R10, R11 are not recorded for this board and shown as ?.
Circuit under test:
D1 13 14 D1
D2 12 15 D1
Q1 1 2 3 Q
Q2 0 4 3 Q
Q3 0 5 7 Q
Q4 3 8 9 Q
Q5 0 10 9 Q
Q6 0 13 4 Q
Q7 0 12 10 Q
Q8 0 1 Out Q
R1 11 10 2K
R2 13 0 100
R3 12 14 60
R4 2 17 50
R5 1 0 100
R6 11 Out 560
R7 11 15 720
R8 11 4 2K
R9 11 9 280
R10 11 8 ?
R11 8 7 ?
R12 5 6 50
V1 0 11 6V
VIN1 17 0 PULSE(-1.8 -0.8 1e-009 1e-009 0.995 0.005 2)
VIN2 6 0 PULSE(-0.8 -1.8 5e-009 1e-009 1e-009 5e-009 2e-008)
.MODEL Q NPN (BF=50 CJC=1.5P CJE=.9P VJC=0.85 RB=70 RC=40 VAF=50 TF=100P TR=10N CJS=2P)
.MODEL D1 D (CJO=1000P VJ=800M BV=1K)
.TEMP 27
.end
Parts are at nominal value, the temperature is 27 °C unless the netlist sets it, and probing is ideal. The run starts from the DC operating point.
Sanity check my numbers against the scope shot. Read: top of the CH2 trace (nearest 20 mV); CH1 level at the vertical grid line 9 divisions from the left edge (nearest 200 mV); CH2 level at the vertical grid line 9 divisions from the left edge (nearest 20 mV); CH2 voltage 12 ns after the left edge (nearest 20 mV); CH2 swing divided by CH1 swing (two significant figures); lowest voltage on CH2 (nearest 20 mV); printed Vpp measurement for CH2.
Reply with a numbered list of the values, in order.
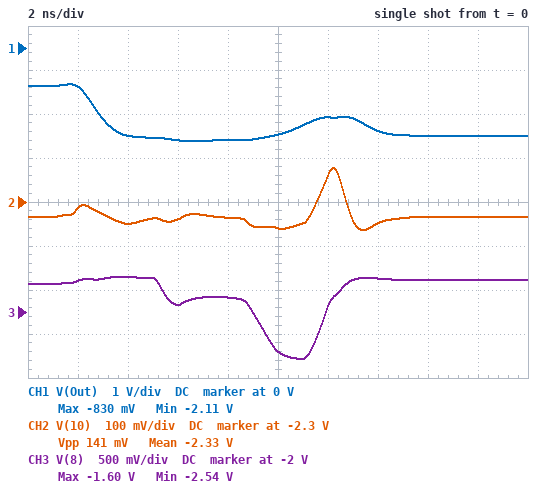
1. -2.22 V
2. -2.0 V
3. -2.34 V
4. -2.24 V
5. 0.11
6. -2.36 V
7. 141 mV
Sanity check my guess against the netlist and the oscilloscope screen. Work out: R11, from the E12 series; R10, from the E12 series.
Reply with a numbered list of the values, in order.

1. 18 Ω
2. 2.2 kΩ
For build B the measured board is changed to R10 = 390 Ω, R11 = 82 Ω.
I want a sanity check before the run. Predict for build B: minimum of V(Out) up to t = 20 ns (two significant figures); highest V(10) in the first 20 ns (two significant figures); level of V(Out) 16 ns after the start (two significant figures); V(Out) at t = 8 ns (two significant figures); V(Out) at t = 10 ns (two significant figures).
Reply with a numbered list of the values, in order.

1. -1.1 V
2. -2.3 V
3. -880 mV
4. -900 mV
5. -870 mV
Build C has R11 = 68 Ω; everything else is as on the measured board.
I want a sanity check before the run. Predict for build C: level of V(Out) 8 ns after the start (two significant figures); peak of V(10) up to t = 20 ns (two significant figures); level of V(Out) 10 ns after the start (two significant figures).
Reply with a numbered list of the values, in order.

1. -1.8 V
2. -2.3 V
3. -1.1 V
